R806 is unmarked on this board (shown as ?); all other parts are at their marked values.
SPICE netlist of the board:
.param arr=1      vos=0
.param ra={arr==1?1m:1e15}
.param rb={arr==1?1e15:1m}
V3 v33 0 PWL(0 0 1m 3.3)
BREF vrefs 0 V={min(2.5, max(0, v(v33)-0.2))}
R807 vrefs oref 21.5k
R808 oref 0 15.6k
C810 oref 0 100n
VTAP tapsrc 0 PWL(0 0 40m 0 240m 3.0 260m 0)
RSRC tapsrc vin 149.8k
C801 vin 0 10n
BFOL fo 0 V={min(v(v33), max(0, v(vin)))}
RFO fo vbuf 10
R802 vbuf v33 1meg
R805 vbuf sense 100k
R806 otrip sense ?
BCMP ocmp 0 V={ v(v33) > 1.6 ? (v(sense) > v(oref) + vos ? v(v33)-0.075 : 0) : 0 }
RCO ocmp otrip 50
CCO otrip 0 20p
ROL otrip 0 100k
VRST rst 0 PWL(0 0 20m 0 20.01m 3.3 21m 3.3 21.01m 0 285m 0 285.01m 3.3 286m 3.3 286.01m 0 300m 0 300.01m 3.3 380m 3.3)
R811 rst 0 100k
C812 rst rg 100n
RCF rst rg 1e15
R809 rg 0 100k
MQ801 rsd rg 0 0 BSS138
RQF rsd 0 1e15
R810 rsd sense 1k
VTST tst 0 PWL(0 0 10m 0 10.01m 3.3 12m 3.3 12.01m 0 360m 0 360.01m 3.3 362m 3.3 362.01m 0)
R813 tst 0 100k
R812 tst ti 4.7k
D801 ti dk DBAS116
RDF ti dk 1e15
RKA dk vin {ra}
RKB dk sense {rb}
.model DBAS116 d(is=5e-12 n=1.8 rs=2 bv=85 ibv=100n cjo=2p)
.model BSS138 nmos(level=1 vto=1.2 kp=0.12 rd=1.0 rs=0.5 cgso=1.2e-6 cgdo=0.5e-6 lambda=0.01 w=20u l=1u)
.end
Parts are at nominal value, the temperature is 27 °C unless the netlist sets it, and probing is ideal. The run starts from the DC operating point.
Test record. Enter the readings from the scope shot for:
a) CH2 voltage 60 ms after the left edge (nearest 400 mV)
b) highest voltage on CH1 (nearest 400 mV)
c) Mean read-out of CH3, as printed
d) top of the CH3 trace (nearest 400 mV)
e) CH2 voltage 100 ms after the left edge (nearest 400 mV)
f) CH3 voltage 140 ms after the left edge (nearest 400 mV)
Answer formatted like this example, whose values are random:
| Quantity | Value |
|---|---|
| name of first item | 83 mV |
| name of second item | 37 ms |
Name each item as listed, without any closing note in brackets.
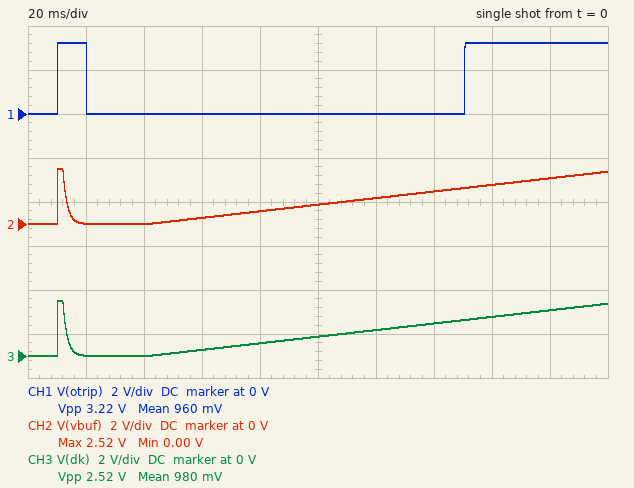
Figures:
| Quantity | Value |
|---|---|
| CH2 voltage 60 ms after the left edge | 400 mV |
| highest voltage on CH1 | 3.2 V |
| Mean read-out of CH3, as printed | 980 mV |
| top of the CH3 trace | 2.4 V |
| CH2 voltage 100 ms after the left edge | 800 mV |
| CH3 voltage 140 ms after the left edge | 1.6 V |
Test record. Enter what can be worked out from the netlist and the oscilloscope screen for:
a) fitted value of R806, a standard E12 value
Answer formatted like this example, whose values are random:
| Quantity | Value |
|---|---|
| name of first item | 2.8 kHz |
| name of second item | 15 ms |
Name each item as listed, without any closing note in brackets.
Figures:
| Quantity | Value |
|---|---|
| fitted value of R806, a standard E12 value | 180 kΩ |
